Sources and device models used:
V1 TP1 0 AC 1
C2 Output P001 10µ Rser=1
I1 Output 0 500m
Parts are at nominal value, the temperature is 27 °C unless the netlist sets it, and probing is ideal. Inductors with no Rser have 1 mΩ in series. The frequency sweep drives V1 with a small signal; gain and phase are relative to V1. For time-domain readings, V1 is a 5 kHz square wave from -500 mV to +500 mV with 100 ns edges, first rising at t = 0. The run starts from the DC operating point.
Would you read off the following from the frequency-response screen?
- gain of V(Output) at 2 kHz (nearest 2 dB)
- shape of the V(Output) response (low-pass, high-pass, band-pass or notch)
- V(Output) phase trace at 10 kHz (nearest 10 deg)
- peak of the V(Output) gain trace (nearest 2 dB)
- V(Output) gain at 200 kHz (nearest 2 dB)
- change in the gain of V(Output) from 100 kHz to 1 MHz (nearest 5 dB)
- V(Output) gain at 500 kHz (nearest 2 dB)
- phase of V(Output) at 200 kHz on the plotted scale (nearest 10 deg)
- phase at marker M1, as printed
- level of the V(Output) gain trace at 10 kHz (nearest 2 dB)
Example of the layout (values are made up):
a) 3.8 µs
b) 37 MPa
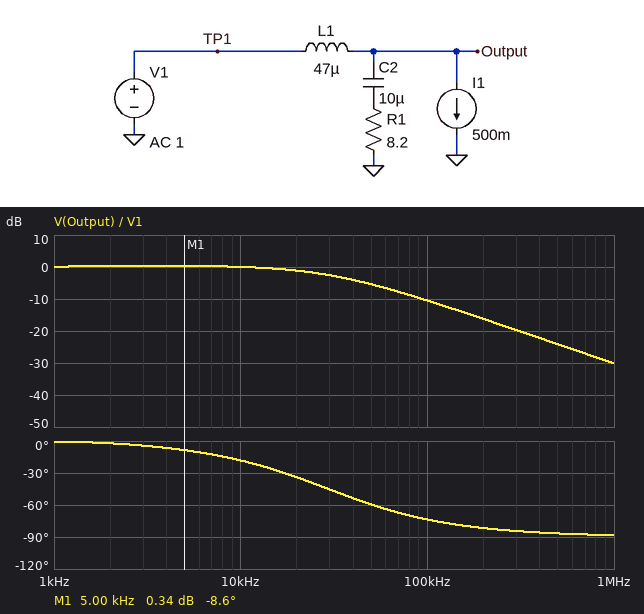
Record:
a) 0 dB
b) low-pass
c) -20 deg
d) 0 dB
e) -16 dB
f) -20 dB
g) -24 dB
h) -80 deg
i) -8.6 deg
j) 0 dB
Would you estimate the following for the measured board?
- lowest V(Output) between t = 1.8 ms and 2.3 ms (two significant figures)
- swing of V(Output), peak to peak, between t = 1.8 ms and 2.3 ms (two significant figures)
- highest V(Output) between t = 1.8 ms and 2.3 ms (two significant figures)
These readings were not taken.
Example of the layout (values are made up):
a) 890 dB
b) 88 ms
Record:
a) -530 mV
b) 1.1 V
c) 530 mV
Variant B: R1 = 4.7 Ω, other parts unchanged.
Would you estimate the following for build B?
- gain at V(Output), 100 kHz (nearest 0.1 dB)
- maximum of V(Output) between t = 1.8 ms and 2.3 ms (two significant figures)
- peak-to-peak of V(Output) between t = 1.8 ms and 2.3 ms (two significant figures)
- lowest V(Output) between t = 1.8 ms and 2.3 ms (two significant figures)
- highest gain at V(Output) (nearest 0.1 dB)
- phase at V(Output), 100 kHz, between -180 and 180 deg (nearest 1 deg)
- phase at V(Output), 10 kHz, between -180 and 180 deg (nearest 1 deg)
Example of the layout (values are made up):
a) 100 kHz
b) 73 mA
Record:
a) -14.4 dB
b) 580 mV
c) 1.2 V
d) -580 mV
e) 0.8 dB
f) -81 deg
g) -29 deg
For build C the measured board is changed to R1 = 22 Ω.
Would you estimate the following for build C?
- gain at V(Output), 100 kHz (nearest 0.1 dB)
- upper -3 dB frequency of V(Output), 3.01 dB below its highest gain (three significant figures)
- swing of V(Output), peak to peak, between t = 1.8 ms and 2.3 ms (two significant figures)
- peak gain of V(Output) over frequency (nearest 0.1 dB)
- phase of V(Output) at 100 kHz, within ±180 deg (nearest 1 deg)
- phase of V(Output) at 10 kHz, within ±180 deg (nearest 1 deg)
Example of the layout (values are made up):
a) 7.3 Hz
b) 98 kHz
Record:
a) -4.2 dB
b) 77.4 kHz
c) 1.0 V
d) 0.1 dB
e) -52 deg
f) -7 deg
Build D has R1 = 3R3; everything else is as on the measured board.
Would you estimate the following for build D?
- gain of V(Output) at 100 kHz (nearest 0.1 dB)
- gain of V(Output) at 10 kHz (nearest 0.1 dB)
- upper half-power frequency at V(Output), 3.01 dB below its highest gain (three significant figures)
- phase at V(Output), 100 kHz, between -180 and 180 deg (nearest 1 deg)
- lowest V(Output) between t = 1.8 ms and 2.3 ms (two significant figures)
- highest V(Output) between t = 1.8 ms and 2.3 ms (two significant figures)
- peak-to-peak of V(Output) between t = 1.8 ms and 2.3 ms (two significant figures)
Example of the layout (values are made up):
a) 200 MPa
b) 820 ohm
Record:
a) -16.8 dB
b) 0.1 dB
c) 14.8 kHz
d) -84 deg
e) -630 mV
f) 630 mV
g) 1.3 V
